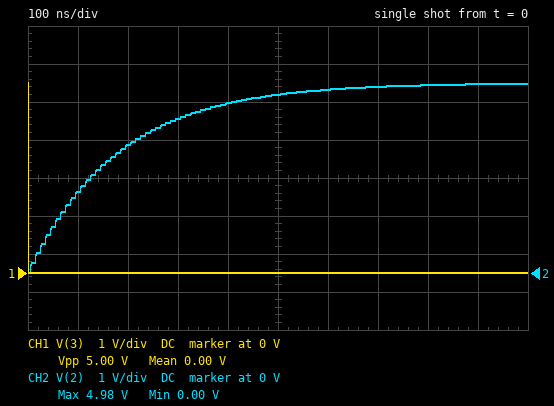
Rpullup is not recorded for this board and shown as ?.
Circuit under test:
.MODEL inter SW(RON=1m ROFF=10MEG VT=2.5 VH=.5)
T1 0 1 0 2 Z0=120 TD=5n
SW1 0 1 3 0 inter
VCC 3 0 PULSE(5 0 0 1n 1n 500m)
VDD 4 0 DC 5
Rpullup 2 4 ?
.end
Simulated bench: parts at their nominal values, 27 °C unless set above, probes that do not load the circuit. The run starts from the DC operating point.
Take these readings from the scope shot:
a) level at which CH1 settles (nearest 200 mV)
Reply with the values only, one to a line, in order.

0 V
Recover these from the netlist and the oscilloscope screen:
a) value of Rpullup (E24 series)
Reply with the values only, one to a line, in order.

4.3 kΩ
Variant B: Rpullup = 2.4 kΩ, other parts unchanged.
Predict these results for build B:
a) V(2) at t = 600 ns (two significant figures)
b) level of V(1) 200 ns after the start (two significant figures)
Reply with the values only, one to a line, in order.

5.0 V
4.3 V
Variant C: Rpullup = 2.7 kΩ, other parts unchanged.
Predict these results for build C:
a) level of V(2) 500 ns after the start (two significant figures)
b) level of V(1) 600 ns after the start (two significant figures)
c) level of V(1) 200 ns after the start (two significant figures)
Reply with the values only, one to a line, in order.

4.9 V
5.0 V
4.1 V
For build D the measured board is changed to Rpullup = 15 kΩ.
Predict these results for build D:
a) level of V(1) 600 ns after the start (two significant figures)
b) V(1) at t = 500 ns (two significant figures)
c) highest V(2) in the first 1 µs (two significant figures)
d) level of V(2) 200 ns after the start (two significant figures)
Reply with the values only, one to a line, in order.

3.1 V
2.7 V
4.0 V
1.4 V
